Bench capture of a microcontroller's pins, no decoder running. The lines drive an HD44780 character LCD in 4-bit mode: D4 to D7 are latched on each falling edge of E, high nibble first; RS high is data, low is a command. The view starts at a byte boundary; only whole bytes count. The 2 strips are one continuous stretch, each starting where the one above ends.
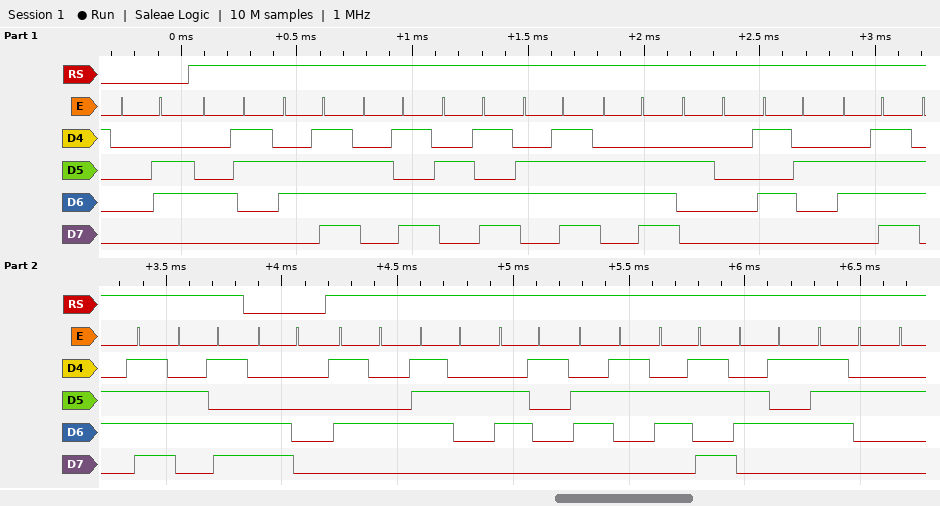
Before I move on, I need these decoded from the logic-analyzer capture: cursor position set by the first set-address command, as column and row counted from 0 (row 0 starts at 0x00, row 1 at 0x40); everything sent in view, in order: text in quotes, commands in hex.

column 0, row 1
0x06 "Common Room" 0xC0 "Tracker"
